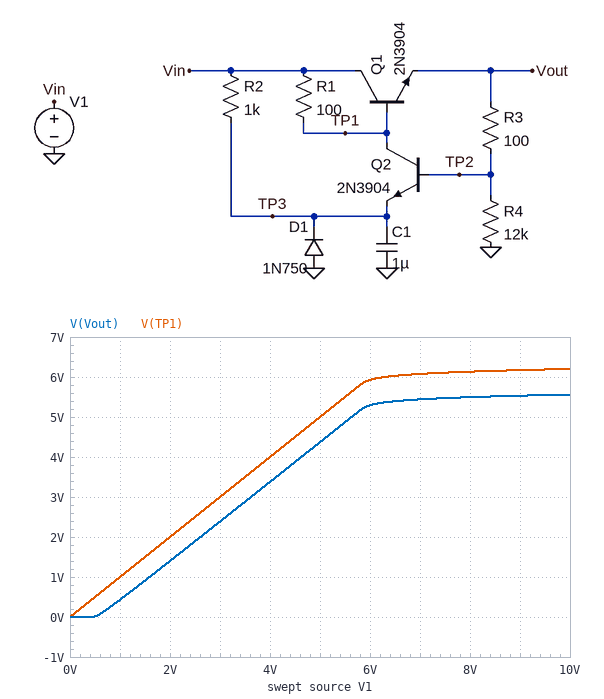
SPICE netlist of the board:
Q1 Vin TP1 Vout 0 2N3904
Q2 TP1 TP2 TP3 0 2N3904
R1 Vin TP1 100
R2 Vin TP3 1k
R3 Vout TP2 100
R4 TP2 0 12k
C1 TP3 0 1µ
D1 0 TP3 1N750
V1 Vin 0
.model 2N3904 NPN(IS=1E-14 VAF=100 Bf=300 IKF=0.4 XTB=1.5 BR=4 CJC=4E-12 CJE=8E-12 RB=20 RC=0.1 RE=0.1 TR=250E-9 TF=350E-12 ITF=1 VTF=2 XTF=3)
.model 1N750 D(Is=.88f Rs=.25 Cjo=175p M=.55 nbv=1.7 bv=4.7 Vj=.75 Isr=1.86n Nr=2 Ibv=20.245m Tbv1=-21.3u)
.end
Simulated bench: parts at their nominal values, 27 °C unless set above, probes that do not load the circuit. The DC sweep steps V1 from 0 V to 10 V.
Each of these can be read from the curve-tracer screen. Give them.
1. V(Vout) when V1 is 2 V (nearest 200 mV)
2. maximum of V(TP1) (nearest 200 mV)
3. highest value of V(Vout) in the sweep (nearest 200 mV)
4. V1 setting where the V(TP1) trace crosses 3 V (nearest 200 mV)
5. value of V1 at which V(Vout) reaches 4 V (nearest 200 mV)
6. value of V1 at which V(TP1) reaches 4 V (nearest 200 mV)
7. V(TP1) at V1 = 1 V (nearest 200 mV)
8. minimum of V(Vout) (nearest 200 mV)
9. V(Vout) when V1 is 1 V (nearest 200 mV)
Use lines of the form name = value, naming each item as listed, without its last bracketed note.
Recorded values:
V(Vout) when V1 is 2 V = 1.4 V
maximum of V(TP1) = 6.2 V
highest value of V(Vout) in the sweep = 5.6 V
V1 setting where the V(TP1) trace crosses 3 V = 3.0 V
value of V1 at which V(Vout) reaches 4 V = 4.6 V
value of V1 at which V(TP1) reaches 4 V = 4.0 V
V(TP1) at V1 = 1 V = 1.0 V
minimum of V(Vout) = 0 V
V(Vout) when V1 is 1 V = 400 mV
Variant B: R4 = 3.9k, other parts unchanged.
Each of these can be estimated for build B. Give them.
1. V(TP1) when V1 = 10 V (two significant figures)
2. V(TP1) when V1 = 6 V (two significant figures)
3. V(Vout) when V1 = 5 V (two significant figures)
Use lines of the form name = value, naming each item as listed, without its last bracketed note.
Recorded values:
V(TP1) when V1 = 10 V = 6.3 V
V(TP1) when V1 = 6 V = 6.0 V
V(Vout) when V1 = 5 V = 4.3 V
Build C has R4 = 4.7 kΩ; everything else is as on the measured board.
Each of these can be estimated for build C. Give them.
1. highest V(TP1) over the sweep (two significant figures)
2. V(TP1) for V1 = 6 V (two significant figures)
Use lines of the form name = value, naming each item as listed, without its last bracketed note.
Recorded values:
highest V(TP1) over the sweep = 6.3 V
V(TP1) for V1 = 6 V = 6.0 V
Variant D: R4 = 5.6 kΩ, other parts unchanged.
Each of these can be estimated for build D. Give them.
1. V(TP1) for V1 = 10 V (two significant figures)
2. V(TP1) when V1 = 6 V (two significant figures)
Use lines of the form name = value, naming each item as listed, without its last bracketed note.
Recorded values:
V(TP1) for V1 = 10 V = 6.3 V
V(TP1) when V1 = 6 V = 6.0 V
